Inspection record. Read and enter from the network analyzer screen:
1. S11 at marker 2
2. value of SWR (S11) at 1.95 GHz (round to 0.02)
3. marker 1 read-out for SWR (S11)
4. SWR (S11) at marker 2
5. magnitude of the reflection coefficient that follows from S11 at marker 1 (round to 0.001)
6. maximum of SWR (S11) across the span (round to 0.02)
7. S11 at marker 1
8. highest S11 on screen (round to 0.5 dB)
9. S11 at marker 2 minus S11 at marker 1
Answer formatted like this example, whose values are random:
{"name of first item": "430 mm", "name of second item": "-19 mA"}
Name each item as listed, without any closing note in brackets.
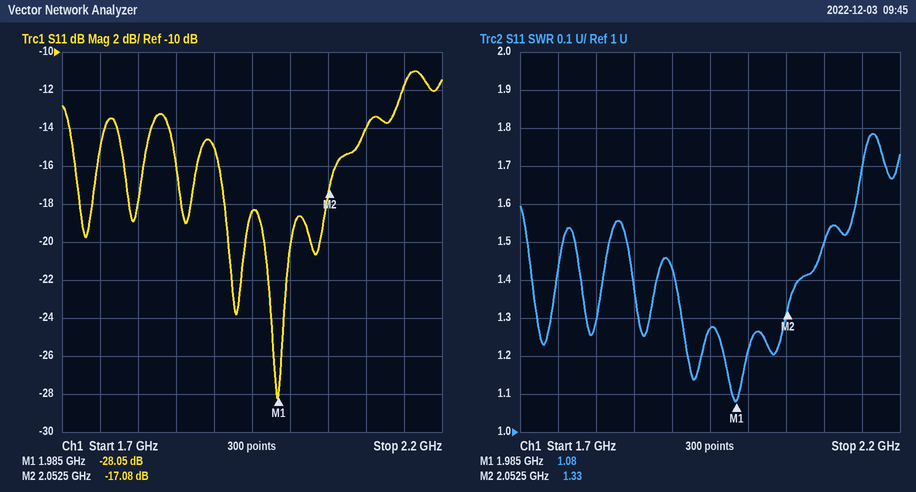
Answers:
{"S11 at marker 2": "-17.08 dB", "value of SWR (S11) at 1.95 GHz": "1.28", "marker 1 read-out for SWR": "1.08", "SWR (S11) at marker 2": "1.33", "magnitude of the reflection coefficient that follows from S11 at marker 1": "0.040", "maximum of SWR (S11) across the span": "1.78", "S11 at marker 1": "-28.05 dB", "highest S11 on screen": "-11.0 dB", "S11 at marker 2 minus S11 at marker 1": "10.97 dB"}
